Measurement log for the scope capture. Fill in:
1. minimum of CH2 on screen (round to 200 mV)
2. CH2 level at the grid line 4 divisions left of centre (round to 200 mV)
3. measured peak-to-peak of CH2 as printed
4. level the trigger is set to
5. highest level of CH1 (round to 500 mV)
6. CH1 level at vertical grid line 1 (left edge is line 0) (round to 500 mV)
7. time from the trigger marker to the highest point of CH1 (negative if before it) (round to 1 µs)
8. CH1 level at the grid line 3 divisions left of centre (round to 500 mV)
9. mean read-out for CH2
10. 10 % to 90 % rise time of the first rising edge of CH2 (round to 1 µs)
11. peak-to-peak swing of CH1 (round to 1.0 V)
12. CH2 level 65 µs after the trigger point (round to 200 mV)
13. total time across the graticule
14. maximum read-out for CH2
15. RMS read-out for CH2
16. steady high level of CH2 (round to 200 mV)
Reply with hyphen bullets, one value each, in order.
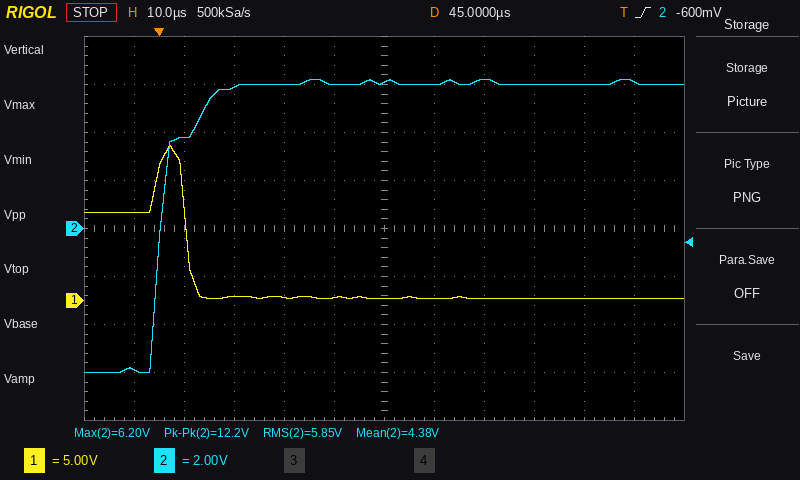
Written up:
- -6.0 V
- 3.8 V
- 12.2 V
- -600 mV
- 16.0 V
- 9.0 V
- +2 µs
- 500 mV
- 4.38 V
- 10 µs
- 16.0 V
- 6.2 V
- 120 µs
- 6.20 V
- 5.85 V
- 6.0 V
